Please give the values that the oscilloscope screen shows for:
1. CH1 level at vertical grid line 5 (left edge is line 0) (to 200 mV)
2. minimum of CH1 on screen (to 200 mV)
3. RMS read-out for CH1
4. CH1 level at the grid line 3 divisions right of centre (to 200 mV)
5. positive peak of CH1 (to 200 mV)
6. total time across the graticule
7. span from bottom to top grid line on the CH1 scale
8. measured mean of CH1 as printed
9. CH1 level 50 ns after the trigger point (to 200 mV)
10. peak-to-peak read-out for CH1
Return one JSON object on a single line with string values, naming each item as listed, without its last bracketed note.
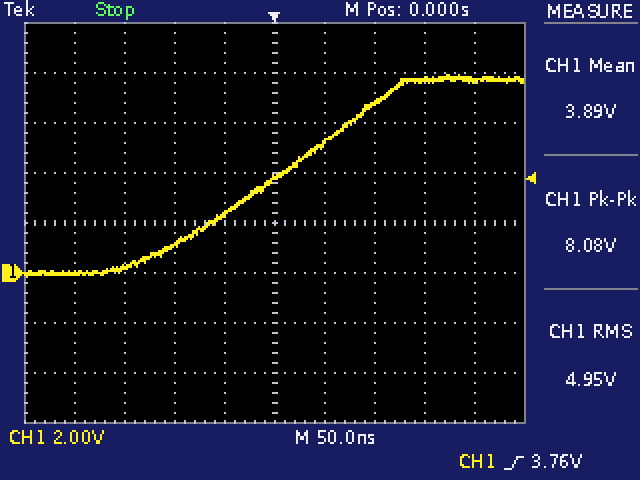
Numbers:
{"CH1 level at vertical grid line 5 (left edge is line 0)": "3.8 V", "minimum of CH1 on screen": "-200 mV", "RMS read-out for CH1": "4.95 V", "CH1 level at the grid line 3 divisions right of centre": "7.8 V", "positive peak of CH1": "8.0 V", "total time across the graticule": "500 ns", "span from bottom to top grid line on the CH1 scale": "16 V", "measured mean of CH1 as printed": "3.89 V", "CH1 level 50 ns after the trigger point": "5.2 V", "peak-to-peak read-out for CH1": "8.08 V"}
